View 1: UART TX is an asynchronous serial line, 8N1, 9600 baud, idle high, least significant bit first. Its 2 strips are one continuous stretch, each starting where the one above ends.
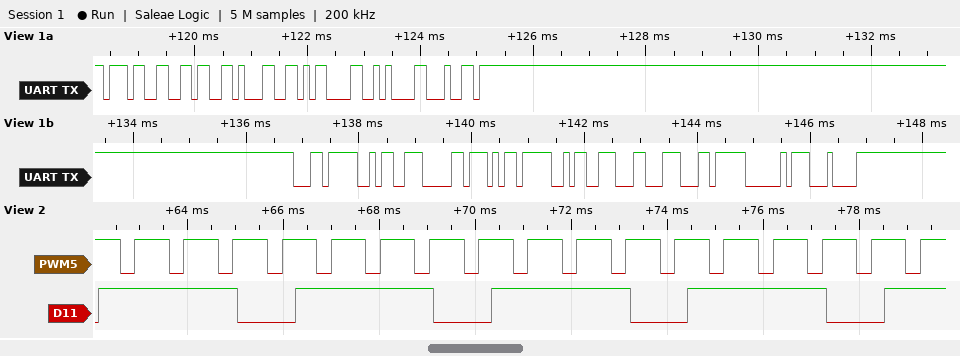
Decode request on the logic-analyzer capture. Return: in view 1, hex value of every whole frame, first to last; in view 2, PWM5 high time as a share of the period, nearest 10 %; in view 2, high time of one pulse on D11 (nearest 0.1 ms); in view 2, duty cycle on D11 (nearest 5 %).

37 36 31 0D 0A 64 EC 9A B0 ED 9A 8C EC A0 84
70 %
2.9 ms
70 %
